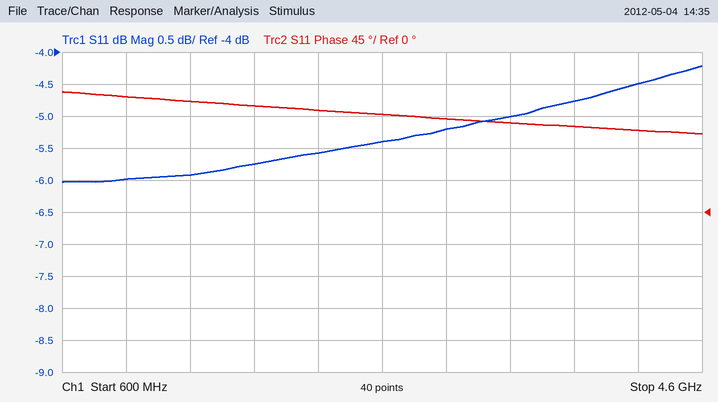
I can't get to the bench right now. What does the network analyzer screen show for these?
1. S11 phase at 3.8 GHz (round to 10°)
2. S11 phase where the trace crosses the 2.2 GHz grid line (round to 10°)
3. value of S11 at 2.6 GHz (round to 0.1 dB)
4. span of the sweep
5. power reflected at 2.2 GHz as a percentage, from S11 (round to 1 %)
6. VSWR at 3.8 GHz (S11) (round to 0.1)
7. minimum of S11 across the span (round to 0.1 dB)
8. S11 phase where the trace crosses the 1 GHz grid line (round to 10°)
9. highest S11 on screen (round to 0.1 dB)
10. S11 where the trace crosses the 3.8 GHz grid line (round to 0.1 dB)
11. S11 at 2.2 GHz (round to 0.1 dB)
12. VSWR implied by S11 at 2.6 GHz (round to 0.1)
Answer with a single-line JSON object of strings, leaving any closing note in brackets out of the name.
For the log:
{"S11 phase at 3.8 GHz": "120°", "S11 phase where the trace crosses the 2.2 GHz grid line": "140°", "value of S11 at 2.6 GHz": "-5.4 dB", "span of the sweep": "4 GHz", "power reflected at 2.2 GHz as a percentage, from S11": "28 %", "VSWR at 3.8 GHz (S11)": "3.7", "minimum of S11 across the span": "-6.0 dB", "S11 phase where the trace crosses the 1 GHz grid line": "160°", "highest S11 on screen": "-4.2 dB", "S11 where the trace crosses the 3.8 GHz grid line": "-4.8 dB", "S11 at 2.2 GHz": "-5.6 dB", "VSWR implied by S11 at 2.6 GHz": "3.3"}
